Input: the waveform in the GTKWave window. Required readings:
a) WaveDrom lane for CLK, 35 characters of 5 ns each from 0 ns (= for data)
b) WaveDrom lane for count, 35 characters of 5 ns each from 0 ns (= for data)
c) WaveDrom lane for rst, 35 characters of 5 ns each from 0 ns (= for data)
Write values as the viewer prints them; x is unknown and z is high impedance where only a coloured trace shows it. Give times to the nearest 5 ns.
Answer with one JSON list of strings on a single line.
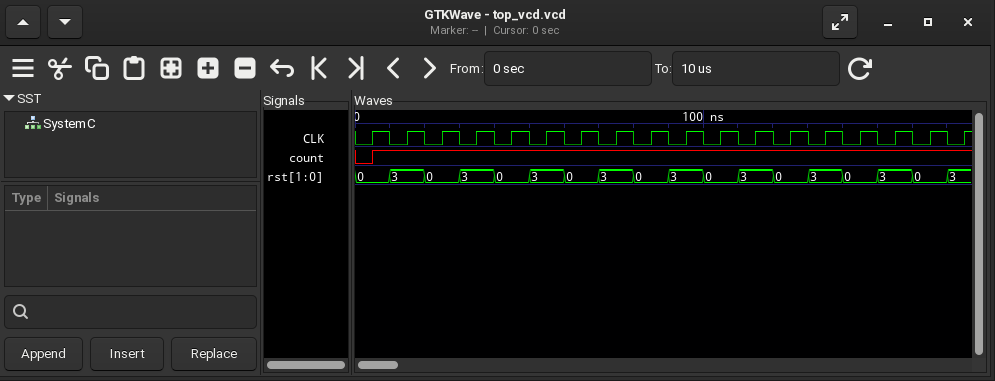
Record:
["{name: 'CLK', wave: '01010101010101010101010101010101010'}", "{name: 'count', wave: '01.................................'}", "{name: 'rst', wave: '=.=.=.=.=.=.=.=.=.=.=.=.=.=.=.=.=.=', data: '0 3 0 3 0 3 0 3 0 3 0 3 0 3 0 3 0 3'}"]
